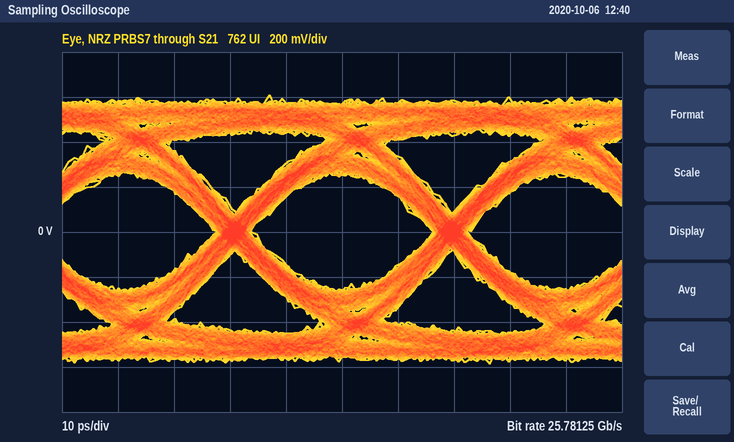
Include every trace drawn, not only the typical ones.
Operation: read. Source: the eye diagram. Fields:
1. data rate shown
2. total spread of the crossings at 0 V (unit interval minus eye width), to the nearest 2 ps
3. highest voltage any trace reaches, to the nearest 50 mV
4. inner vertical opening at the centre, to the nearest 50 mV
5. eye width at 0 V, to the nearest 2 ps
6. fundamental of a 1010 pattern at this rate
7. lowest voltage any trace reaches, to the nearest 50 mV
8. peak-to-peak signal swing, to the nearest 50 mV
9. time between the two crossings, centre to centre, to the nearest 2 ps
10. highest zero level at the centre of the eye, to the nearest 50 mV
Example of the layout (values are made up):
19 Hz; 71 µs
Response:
25.78125 Gb/s; 6 ps; 600 mV; 500 mV; 32 ps; 12.89062 GHz; -600 mV; 1.20 V; 38 ps; -250 mV
